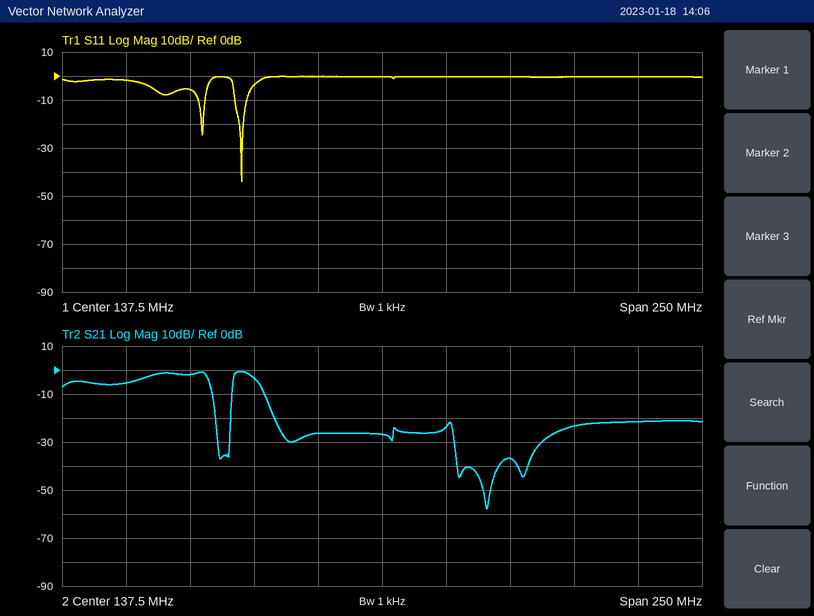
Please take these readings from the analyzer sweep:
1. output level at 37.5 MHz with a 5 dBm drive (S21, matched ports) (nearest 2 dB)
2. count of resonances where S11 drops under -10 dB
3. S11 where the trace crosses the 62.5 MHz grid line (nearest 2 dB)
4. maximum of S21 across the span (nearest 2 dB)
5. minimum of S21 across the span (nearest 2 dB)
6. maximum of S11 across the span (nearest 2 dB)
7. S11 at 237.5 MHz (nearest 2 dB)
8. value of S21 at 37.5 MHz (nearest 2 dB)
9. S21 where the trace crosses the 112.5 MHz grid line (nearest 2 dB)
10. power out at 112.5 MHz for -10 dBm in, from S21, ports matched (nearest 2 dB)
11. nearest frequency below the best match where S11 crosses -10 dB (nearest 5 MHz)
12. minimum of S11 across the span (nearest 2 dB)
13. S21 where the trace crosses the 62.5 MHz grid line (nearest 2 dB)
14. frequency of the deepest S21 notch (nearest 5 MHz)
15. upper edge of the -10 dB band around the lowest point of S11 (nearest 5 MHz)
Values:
0 dBm
2
-6 dB
0 dB
-58 dB
0 dB
0 dB
-6 dB
-26 dB
-36 dBm
80 MHz
-44 dB
-2 dB
180 MHz
85 MHz
